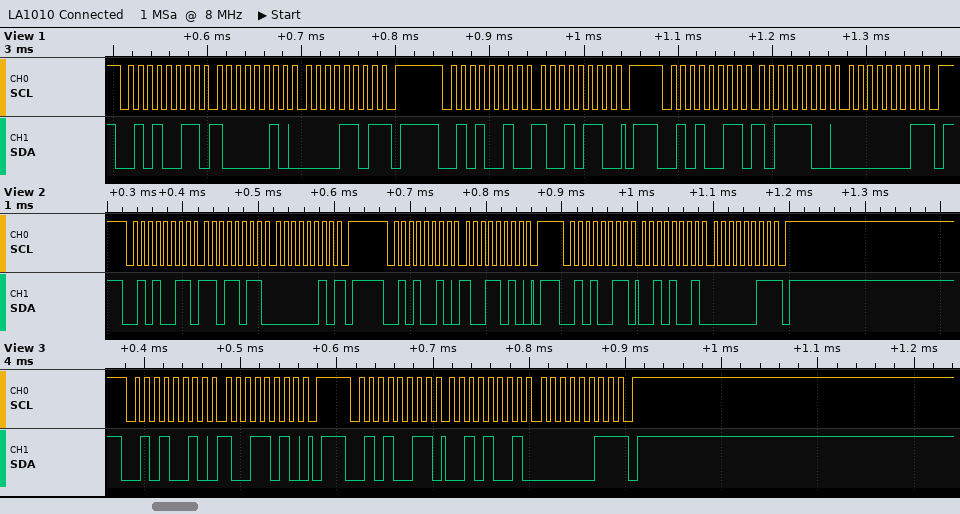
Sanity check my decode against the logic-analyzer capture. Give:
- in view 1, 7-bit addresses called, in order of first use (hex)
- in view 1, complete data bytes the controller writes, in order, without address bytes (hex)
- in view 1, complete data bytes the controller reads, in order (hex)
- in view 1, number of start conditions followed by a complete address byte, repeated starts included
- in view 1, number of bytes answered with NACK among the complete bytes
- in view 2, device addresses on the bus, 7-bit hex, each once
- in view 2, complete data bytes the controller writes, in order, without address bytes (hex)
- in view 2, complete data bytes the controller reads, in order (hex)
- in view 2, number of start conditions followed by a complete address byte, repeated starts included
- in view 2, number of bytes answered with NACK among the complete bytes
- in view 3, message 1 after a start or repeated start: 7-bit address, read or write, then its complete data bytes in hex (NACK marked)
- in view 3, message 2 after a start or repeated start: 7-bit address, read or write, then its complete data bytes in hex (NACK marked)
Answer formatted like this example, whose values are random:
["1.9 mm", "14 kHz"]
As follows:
["0x29", "96", "82 0D BC 01", "3", "2", "0x29", "9A", "DB 02 29 03", "3", "2", "0x29 write: 9A", "0x29 read: 29 03 NACK"]
